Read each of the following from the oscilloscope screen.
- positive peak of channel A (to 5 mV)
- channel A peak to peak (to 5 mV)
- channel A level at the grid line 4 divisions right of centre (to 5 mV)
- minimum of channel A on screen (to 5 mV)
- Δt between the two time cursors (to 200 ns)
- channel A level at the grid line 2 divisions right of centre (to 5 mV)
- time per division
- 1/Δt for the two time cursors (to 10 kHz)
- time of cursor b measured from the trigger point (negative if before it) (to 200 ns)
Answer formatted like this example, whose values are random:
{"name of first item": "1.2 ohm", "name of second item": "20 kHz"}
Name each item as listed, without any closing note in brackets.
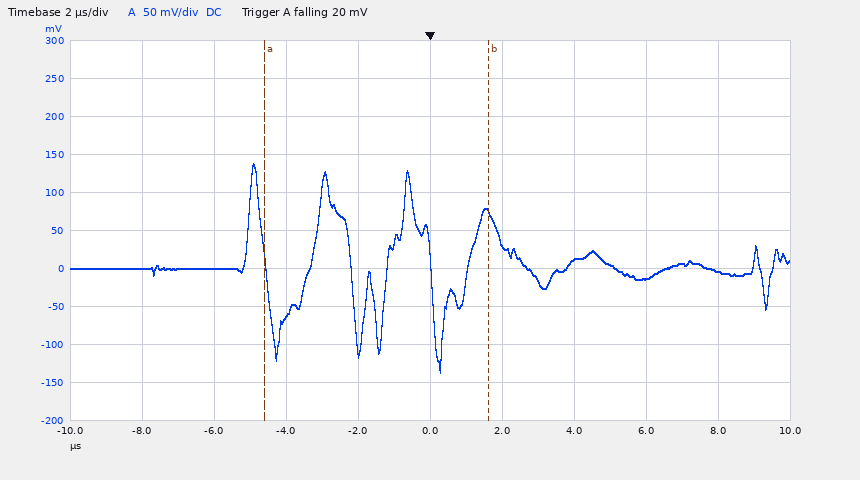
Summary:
{"positive peak of channel A": "140 mV", "channel A peak to peak": "275 mV", "channel A level at the grid line 4 divisions right of centre": "-5 mV", "minimum of channel A on screen": "-135 mV", "Δt between the two time cursors": "6.2 µs", "channel A level at the grid line 2 divisions right of centre": "10 mV", "time per division": "2 µs", "1/Δt for the two time cursors": "160 kHz", "time of cursor b measured from the trigger point (negative if before it)": "+1.6 µs"}
